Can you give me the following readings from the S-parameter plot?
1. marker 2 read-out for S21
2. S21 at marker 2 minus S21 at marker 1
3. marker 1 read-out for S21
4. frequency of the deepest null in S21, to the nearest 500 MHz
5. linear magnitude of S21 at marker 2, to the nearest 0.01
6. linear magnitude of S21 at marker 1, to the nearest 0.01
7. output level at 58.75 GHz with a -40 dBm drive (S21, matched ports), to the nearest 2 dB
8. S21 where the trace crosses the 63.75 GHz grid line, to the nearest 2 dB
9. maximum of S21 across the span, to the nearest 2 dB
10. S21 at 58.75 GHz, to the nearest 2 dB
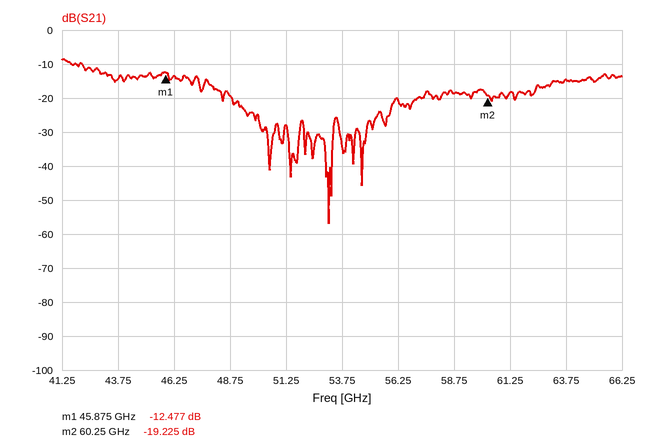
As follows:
-19.225 dB
-6.748 dB
-12.477 dB
53.0 GHz
0.11
0.24
-58 dBm
-14 dB
-8 dB
-18 dB
